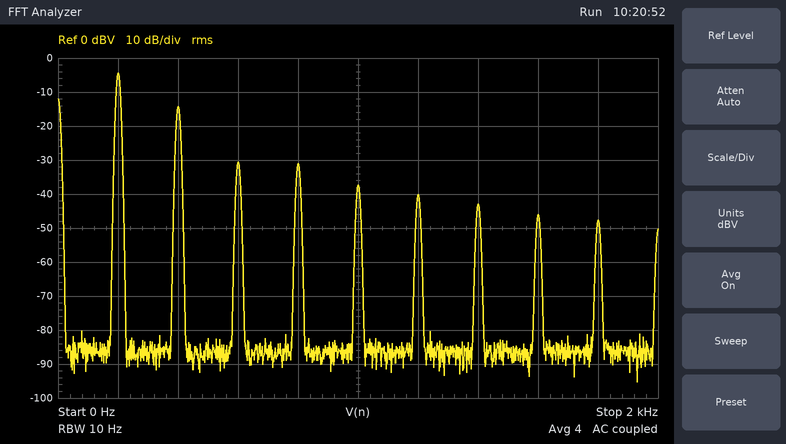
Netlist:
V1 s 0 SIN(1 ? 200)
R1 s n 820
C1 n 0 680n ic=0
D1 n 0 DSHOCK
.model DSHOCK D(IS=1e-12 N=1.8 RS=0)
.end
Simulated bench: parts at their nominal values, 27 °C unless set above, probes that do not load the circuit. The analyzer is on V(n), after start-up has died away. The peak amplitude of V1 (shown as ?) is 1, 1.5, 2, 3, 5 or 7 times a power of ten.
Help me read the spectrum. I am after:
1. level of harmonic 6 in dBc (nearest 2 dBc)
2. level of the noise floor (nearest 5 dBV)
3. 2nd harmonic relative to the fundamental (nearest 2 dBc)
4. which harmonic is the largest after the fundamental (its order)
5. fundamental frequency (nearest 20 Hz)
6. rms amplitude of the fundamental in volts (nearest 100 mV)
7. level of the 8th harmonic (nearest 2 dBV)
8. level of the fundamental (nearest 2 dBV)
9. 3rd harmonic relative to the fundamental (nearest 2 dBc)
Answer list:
-36 dBc
-85 dBV
-10 dBc
2
200 Hz
600 mV
-46 dBV
-4 dBV
-26 dBc
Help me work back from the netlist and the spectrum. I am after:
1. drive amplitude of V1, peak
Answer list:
2 V
